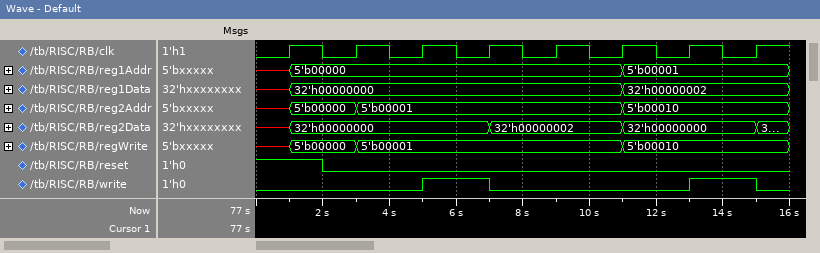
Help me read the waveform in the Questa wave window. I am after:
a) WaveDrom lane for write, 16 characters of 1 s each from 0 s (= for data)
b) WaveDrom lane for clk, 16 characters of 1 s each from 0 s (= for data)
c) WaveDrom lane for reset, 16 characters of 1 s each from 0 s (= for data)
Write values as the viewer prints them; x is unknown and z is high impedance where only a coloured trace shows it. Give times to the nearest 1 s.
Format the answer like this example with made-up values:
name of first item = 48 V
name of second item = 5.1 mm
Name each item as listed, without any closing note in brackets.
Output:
WaveDrom lane for write, 16 characters of 1 s each from 0 s = {name: 'write', wave: '0....1.0.....1.0'}
WaveDrom lane for clk, 16 characters of 1 s each from 0 s = {name: 'clk', wave: '0101010101010101'}
WaveDrom lane for reset, 16 characters of 1 s each from 0 s = {name: 'reset', wave: '1.0.............'}
